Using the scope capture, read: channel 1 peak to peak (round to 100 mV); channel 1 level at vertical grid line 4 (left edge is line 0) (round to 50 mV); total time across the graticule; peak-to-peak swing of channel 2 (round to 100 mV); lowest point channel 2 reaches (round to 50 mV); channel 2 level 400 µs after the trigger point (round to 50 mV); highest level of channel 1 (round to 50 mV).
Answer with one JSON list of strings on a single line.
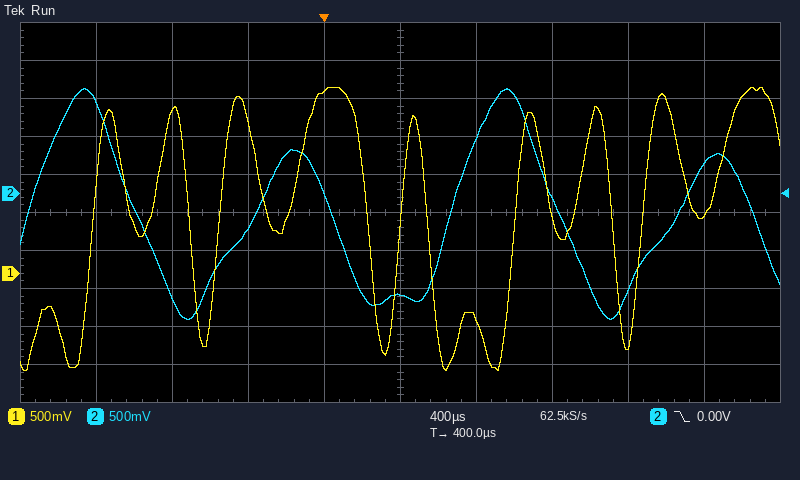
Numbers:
["3.70 V", "2.40 V", "4 ms", "3.00 V", "-1.65 V", "-1.35 V", "2.45 V"]
